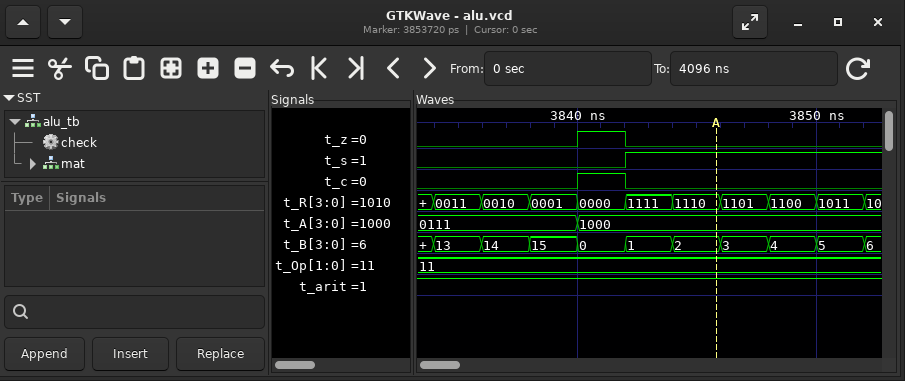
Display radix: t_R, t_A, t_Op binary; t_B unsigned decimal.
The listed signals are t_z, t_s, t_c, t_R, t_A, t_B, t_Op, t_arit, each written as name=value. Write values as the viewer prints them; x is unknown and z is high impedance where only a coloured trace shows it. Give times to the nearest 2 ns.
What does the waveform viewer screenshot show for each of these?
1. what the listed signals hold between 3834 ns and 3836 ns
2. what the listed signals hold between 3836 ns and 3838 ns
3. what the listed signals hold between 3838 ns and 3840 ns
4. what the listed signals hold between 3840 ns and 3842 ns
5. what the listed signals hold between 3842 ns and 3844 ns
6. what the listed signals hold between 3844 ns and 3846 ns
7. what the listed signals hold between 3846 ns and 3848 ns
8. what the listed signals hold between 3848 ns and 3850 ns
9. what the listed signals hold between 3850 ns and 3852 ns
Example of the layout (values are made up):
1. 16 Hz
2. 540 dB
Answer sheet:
1. t_z=0, t_s=0, t_c=0, t_R=0011, t_A=0111, t_B=13, t_Op=11, t_arit=1
2. t_z=0, t_s=0, t_c=0, t_R=0010, t_A=0111, t_B=14, t_Op=11, t_arit=1
3. t_z=0, t_s=0, t_c=0, t_R=0001, t_A=0111, t_B=15, t_Op=11, t_arit=1
4. t_z=1, t_s=0, t_c=1, t_R=0000, t_A=1000, t_B=0, t_Op=11, t_arit=1
5. t_z=0, t_s=1, t_c=0, t_R=1111, t_A=1000, t_B=1, t_Op=11, t_arit=1
6. t_z=0, t_s=1, t_c=0, t_R=1110, t_A=1000, t_B=2, t_Op=11, t_arit=1
7. t_z=0, t_s=1, t_c=0, t_R=1101, t_A=1000, t_B=3, t_Op=11, t_arit=1
8. t_z=0, t_s=1, t_c=0, t_R=1100, t_A=1000, t_B=4, t_Op=11, t_arit=1
9. t_z=0, t_s=1, t_c=0, t_R=1011, t_A=1000, t_B=5, t_Op=11, t_arit=1
